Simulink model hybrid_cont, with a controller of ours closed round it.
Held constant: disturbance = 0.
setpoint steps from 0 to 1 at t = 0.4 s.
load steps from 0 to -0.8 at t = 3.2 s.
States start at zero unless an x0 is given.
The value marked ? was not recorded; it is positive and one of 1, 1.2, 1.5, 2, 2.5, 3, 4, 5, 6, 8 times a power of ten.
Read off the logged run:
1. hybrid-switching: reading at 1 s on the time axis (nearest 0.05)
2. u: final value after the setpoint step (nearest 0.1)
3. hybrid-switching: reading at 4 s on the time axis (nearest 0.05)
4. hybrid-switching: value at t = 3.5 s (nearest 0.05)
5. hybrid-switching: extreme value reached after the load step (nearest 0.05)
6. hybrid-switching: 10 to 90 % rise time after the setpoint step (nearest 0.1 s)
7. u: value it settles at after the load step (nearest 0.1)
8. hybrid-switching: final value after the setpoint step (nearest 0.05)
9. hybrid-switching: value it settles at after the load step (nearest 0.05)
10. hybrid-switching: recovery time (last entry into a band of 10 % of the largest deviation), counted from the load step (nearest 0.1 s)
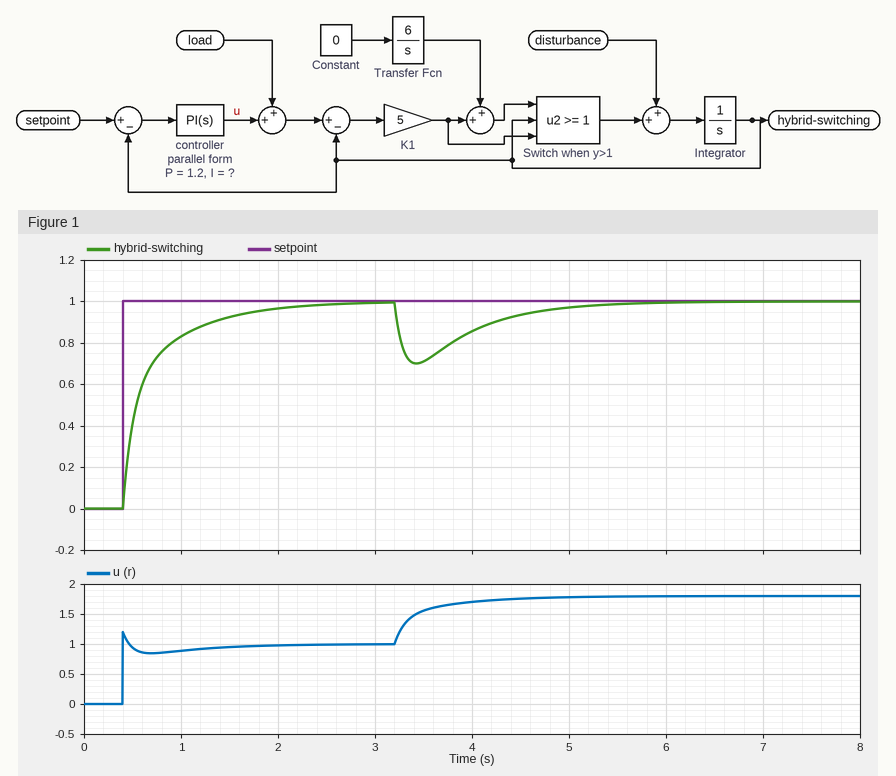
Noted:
0.85
1.0
0.85
0.70
0.70
0.9 s
1.8
1.00
1.00
1.8 s
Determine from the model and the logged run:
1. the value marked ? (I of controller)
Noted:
3
